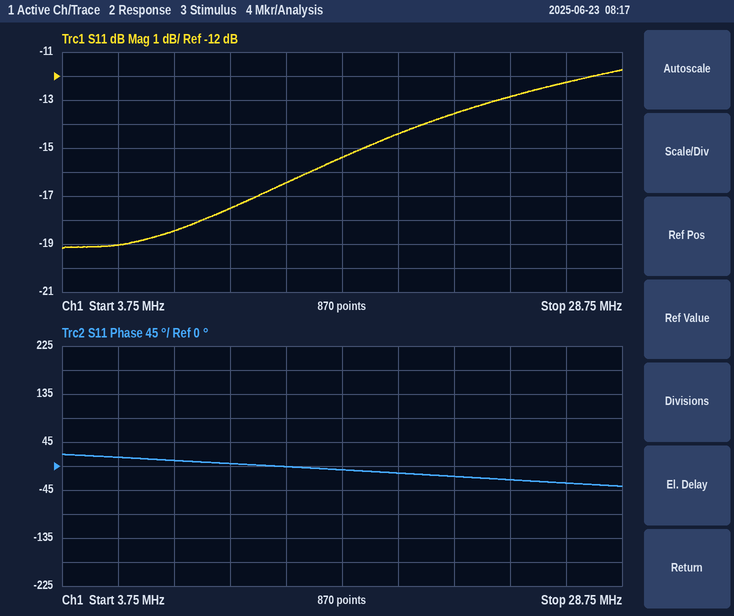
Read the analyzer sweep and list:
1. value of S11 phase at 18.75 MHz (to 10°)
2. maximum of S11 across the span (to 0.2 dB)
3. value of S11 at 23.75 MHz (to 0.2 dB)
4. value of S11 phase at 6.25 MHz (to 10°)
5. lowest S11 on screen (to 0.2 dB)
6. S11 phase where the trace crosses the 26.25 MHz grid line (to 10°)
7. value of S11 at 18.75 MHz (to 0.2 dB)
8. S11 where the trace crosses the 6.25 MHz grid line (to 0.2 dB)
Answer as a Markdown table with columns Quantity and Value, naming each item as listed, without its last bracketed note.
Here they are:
| Quantity | Value |
|---|---|
| value of S11 phase at 18.75 MHz | -10° |
| maximum of S11 across the span | -11.8 dB |
| value of S11 at 23.75 MHz | -12.8 dB |
| value of S11 phase at 6.25 MHz | 20° |
| lowest S11 on screen | -19.2 dB |
| S11 phase where the trace crosses the 26.25 MHz grid line | -30° |
| value of S11 at 18.75 MHz | -14.4 dB |
| S11 where the trace crosses the 6.25 MHz grid line | -19.0 dB |
